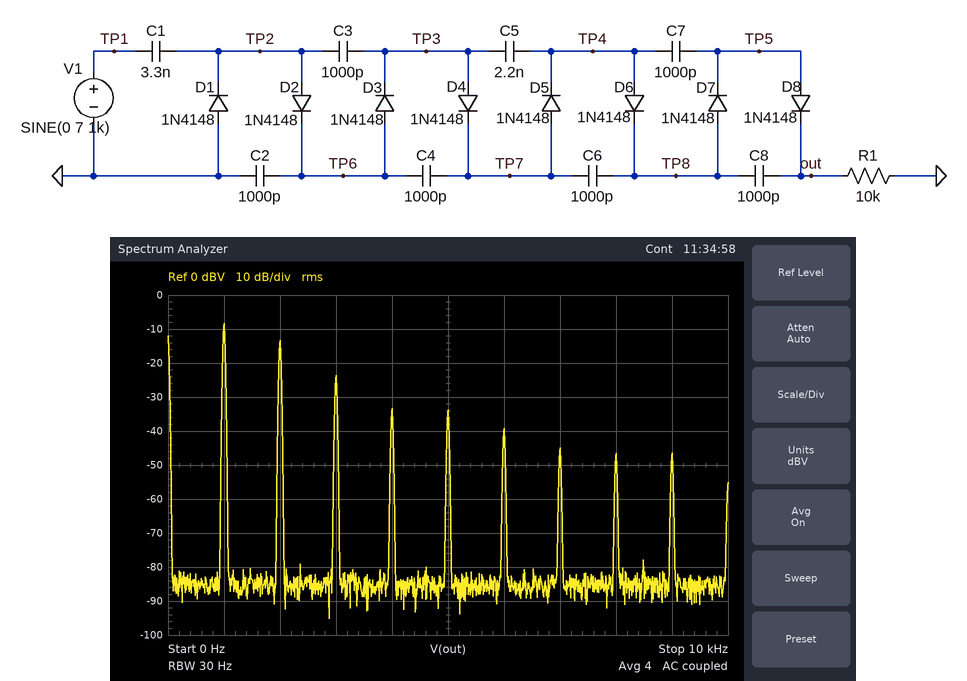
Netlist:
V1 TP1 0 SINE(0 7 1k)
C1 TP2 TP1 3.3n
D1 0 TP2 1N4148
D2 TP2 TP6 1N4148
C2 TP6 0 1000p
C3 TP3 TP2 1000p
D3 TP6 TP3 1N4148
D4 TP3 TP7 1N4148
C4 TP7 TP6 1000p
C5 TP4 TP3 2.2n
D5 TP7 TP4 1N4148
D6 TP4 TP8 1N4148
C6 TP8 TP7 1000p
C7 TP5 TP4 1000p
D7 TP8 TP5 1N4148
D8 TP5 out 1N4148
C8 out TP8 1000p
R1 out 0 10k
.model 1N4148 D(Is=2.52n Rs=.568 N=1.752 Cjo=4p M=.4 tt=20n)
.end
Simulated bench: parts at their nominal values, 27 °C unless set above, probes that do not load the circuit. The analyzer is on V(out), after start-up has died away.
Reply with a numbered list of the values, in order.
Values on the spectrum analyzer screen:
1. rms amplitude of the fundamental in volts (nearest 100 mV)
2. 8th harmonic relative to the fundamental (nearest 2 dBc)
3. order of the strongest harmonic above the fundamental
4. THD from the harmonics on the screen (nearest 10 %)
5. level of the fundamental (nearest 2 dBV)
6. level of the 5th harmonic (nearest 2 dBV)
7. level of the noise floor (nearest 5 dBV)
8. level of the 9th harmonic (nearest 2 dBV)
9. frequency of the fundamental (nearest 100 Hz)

1. 400 mV
2. -38 dBc
3. 2
4. 60 %
5. -8 dBV
6. -34 dBV
7. -85 dBV
8. -46 dBV
9. 1.0 kHz
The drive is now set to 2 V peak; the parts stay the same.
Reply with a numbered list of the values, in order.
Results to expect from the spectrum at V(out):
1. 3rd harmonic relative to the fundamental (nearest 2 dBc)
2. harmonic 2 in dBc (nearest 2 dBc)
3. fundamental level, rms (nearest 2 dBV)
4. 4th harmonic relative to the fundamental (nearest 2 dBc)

1. -26 dBc
2. -10 dBc
3. -30 dBV
4. -28 dBc
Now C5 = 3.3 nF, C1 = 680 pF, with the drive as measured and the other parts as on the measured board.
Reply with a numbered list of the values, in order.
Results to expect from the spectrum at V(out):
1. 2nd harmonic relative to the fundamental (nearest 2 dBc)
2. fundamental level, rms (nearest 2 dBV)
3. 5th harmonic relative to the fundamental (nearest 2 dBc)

1. -6 dBc
2. -22 dBV
3. -24 dBc
